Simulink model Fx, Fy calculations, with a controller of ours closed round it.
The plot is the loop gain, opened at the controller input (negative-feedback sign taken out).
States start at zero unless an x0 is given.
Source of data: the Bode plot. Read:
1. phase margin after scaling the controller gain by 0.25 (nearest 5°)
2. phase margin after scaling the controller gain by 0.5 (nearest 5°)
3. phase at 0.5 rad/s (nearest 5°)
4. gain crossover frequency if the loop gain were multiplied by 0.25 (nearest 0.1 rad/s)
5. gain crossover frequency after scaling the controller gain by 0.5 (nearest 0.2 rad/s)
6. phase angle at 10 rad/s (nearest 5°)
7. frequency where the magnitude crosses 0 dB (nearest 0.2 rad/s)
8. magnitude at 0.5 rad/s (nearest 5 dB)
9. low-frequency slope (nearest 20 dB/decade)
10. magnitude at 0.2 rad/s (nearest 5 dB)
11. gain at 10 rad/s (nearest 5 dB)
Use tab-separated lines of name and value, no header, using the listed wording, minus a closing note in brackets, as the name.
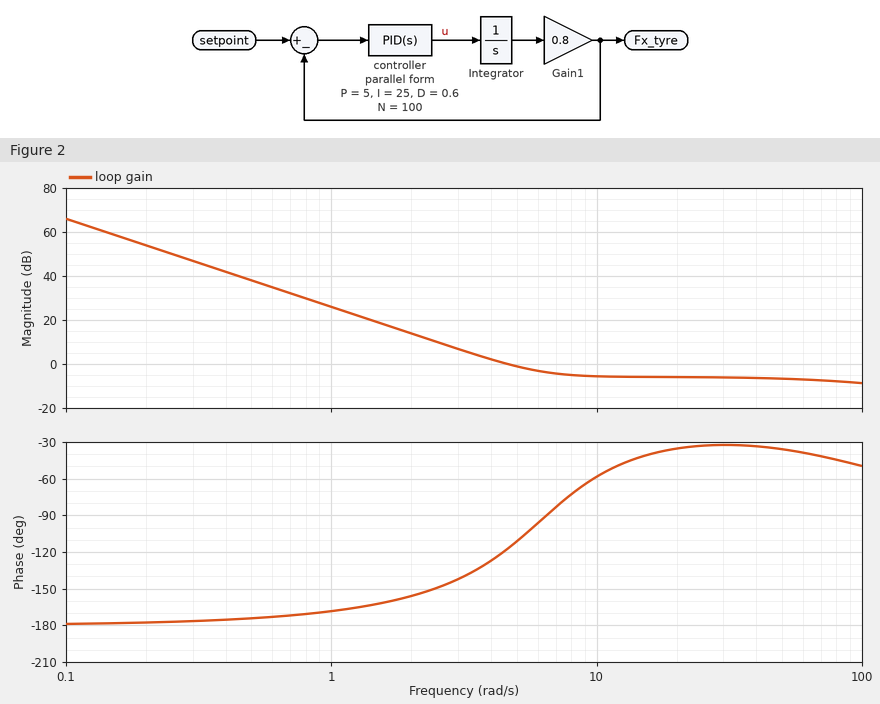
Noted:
phase margin after scaling the controller gain by 0.25	25°
phase margin after scaling the controller gain by 0.5	40°
phase at 0.5 rad/s	-175°
gain crossover frequency if the loop gain were multiplied by 0.25	2.2 rad/s
gain crossover frequency after scaling the controller gain by 0.5	3.2 rad/s
phase angle at 10 rad/s	-60°
frequency where the magnitude crosses 0 dB	4.6 rad/s
magnitude at 0.5 rad/s	40 dB
low-frequency slope	-40 dB/decade
magnitude at 0.2 rad/s	55 dB
gain at 10 rad/s	-5 dB
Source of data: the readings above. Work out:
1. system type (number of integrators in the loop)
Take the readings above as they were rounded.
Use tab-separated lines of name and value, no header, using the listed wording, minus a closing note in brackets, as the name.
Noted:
system type	2
